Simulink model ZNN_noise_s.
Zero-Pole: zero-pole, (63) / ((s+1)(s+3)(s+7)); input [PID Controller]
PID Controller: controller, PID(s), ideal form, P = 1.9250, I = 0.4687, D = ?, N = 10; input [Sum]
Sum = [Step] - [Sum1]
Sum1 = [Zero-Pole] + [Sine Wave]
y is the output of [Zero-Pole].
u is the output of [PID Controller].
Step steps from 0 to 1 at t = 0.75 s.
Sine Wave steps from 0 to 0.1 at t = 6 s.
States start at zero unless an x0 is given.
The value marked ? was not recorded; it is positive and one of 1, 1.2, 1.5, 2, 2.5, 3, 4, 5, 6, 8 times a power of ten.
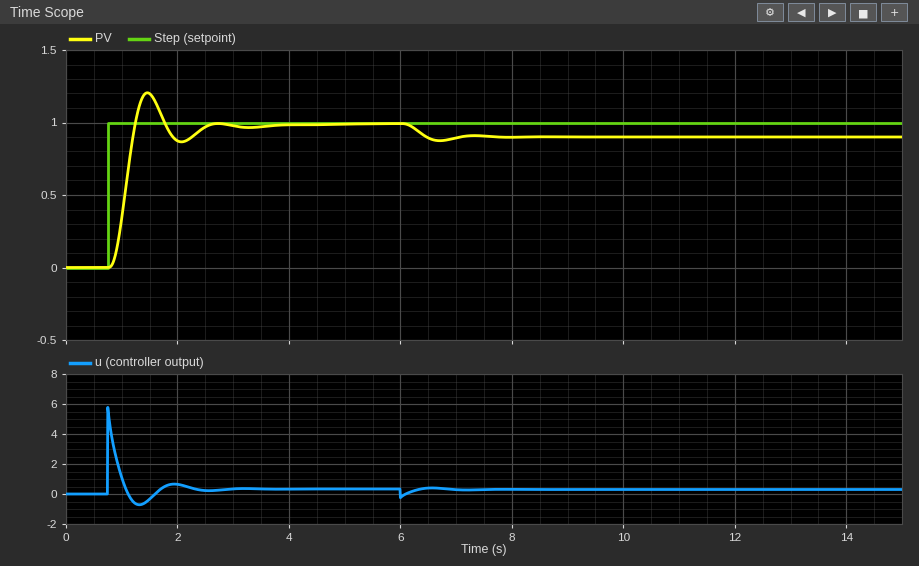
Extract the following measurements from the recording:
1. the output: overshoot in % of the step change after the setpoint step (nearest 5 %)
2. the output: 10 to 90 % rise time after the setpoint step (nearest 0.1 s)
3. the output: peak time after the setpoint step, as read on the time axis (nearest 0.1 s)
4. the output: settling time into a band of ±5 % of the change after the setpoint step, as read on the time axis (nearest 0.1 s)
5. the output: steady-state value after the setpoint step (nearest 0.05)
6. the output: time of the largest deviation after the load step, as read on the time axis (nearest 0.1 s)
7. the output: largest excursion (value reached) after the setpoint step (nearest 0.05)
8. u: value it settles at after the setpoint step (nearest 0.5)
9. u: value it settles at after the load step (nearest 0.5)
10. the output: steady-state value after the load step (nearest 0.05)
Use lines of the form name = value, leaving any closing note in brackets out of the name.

the output: overshoot in % of the step change after the setpoint step = 20 %
the output: 10 to 90 % rise time after the setpoint step = 0.3 s
the output: peak time after the setpoint step, as read on the time axis = 1.5 s
the output: settling time into a band of ±5 % of the change after the setpoint step, as read on the time axis = 2.4 s
the output: steady-state value after the setpoint step = 1.00
the output: time of the largest deviation after the load step, as read on the time axis = 6.7 s
the output: largest excursion (value reached) after the setpoint step = 1.20
u: value it settles at after the setpoint step = 0.5
u: value it settles at after the load step = 0.5
the output: steady-state value after the load step = 0.90
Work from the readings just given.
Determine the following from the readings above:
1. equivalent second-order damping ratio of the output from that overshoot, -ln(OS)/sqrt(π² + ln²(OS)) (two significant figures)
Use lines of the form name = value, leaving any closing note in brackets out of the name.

equivalent second-order damping ratio of the output from that overshoot, -ln(OS)/sqrt(π² + ln²(OS)) = 0.46
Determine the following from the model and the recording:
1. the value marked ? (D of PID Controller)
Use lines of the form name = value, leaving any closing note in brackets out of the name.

the value marked ? = 0.2
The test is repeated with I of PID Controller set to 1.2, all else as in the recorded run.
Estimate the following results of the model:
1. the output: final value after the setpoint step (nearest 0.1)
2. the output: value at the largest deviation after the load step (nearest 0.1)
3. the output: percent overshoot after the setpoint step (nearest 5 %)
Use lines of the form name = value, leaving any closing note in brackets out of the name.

the output: final value after the setpoint step = 1.0
the output: value at the largest deviation after the load step = 0.9
the output: percent overshoot after the setpoint step = 35 %
